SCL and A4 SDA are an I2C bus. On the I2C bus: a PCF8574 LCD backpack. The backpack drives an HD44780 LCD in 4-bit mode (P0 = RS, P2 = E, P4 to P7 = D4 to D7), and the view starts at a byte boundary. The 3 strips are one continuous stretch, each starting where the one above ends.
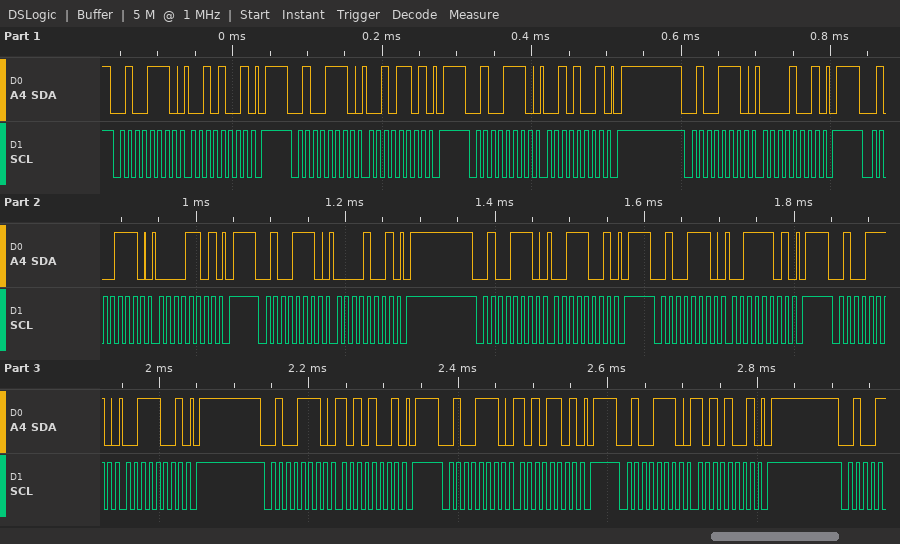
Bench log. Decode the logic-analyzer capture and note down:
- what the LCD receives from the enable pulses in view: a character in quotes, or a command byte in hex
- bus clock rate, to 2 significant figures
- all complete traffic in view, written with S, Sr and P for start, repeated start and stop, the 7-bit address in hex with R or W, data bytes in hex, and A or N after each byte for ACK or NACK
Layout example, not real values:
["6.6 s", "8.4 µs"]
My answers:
["' ' ':'", "100 kHz", "S 27W A 29 A P S 27W A 2D A P S 27W A 29 A P S 27W A 09 A P S 27W A 0D A P S 27W A 09 A P S 27W A 39 A P S 27W A 3D A P S 27W A 39 A P S 27W A A9 A P S 27W A AD A P S 27W A A9 A P"]
